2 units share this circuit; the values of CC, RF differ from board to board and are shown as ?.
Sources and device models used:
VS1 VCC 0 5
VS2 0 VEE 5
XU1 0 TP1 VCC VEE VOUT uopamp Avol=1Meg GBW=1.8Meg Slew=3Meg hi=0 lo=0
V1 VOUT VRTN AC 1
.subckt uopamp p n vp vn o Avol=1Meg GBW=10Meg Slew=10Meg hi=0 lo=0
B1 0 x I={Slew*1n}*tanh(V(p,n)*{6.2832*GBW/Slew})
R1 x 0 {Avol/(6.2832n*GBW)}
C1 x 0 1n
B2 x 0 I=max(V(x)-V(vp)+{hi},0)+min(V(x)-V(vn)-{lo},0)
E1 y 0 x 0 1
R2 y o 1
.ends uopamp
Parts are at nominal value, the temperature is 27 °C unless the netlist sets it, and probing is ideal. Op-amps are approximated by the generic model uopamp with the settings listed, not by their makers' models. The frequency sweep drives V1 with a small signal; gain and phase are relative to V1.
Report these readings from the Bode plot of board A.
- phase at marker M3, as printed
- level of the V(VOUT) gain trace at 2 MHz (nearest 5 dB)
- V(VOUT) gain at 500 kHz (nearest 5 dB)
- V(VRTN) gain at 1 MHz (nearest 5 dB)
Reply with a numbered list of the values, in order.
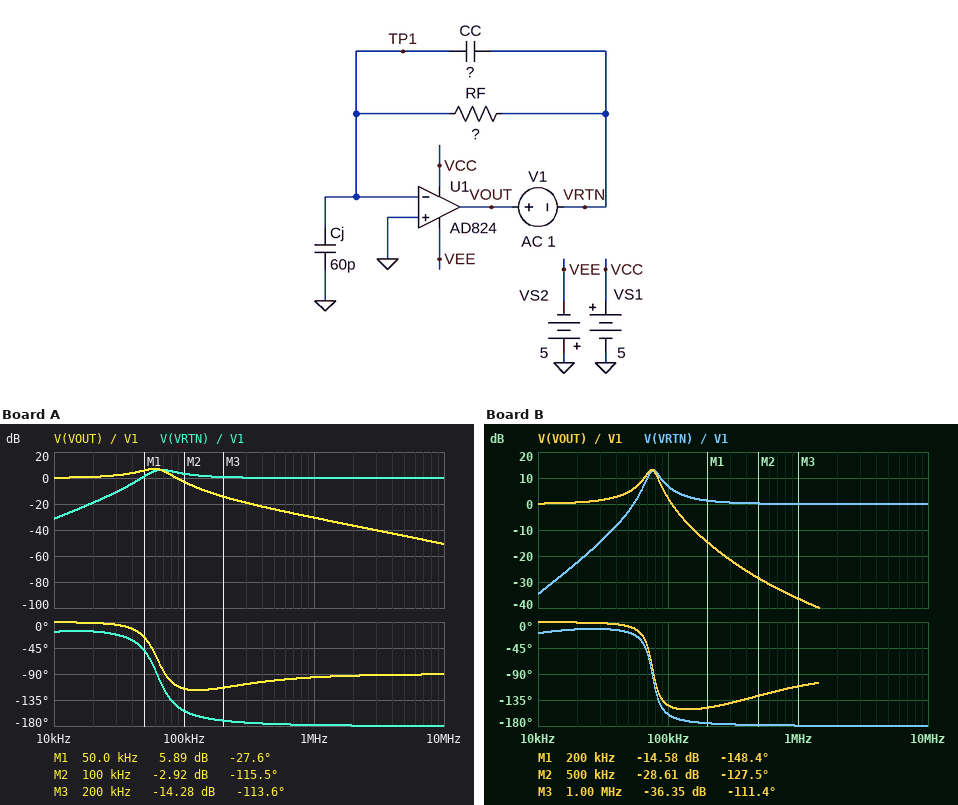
1. -113.6 deg
2. -35 dB
3. -25 dB
4. 0 dB
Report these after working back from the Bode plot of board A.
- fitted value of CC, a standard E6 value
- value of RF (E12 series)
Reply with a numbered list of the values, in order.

1. 1 pF
2. 1.2 MΩ
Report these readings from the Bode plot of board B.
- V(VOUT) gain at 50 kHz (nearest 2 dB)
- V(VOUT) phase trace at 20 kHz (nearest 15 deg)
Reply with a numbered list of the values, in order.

1. 4 dB
2. 0 deg
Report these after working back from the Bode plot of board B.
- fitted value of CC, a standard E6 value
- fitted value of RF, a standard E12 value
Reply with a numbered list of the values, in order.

1. 470 fF
2. 820 kΩ
